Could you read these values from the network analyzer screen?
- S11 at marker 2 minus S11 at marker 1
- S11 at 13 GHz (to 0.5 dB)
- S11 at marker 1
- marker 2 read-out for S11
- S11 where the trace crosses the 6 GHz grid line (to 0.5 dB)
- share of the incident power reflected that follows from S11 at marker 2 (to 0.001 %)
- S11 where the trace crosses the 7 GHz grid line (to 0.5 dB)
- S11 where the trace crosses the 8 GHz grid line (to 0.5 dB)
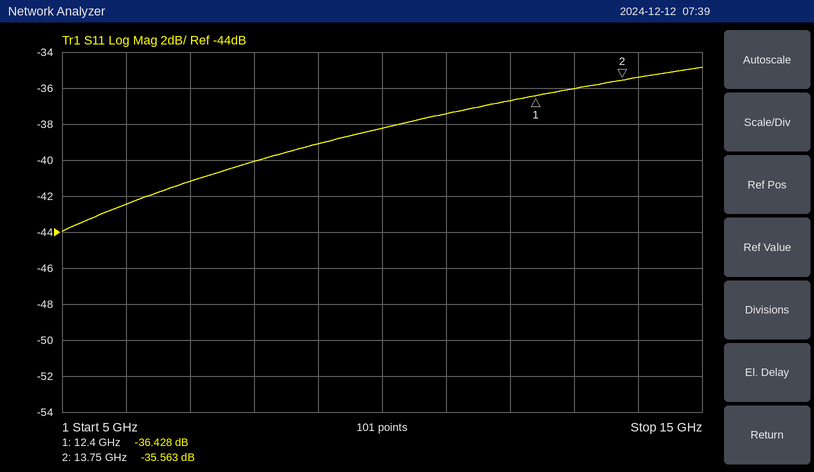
0.865 dB
-36.0 dB
-36.428 dB
-35.563 dB
-42.5 dB
0.028 %
-41.0 dB
-40.0 dB
